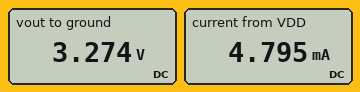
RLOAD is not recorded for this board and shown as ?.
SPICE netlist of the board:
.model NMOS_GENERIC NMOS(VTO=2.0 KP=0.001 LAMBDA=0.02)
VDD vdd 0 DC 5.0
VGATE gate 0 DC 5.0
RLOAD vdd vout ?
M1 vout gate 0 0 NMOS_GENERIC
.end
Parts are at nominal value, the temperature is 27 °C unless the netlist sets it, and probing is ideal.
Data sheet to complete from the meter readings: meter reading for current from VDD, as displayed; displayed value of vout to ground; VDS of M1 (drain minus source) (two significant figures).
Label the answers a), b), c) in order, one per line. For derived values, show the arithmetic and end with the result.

a) 4.795 mA
b) 3.274 V
c) 3.274 V = 3.3 V
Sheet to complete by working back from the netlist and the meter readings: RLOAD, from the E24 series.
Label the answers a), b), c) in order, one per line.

a) 360 Ω
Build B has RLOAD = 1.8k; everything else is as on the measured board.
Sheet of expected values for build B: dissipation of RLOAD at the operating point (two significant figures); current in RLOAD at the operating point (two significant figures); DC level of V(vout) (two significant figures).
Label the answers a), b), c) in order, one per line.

a) 9.4 mW
b) 2.3 mA
c) 880 mV
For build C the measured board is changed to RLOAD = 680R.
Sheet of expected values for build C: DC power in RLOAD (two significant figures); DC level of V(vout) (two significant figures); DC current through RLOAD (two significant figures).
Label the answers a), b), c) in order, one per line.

a) 12 mW
b) 2.1 V
c) 4.3 mA
